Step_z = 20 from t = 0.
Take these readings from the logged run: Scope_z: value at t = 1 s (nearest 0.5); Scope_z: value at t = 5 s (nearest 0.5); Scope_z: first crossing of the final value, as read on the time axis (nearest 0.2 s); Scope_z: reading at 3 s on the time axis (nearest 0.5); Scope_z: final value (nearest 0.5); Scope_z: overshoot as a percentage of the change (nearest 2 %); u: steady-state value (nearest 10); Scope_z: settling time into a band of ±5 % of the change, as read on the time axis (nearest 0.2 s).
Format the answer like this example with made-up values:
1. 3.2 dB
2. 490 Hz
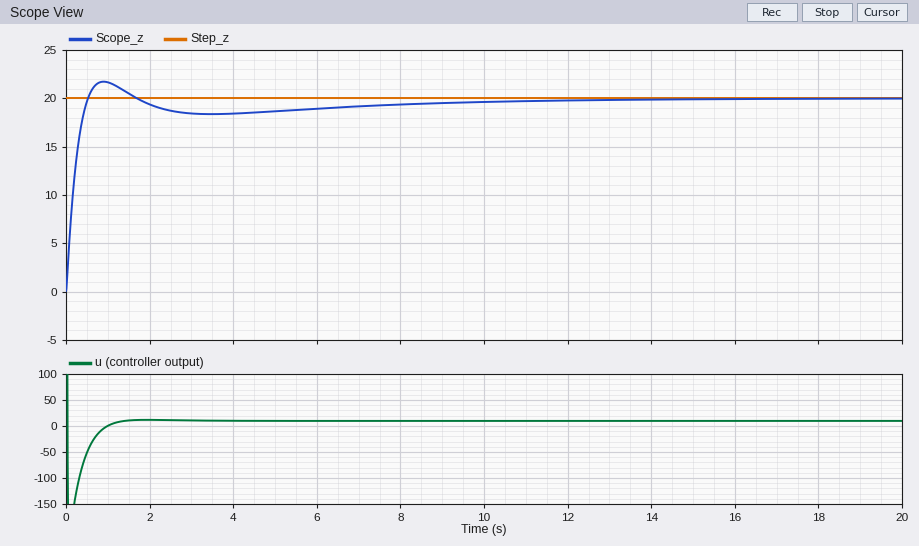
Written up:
1. 21.5
2. 18.5
3. 0.6 s
4. 18.5
5. 20.0
6. 8 %
7. 10
8. 6.2 s
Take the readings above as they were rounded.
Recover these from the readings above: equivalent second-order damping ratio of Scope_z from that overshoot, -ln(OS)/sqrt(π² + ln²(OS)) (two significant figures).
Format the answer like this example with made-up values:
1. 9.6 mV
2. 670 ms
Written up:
1. 0.63
